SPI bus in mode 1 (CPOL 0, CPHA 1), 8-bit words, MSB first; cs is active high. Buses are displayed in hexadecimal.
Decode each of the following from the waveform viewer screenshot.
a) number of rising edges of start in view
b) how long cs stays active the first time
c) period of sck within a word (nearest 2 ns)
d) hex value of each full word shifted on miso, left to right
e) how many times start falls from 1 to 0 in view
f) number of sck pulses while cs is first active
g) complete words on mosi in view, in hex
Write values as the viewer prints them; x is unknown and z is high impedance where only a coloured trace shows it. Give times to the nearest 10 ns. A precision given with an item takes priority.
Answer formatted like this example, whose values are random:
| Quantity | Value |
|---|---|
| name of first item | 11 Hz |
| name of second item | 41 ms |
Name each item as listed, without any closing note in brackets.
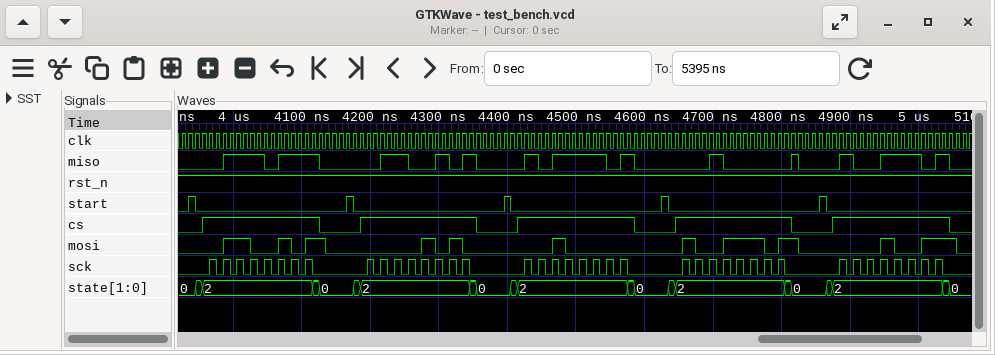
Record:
| Quantity | Value |
|---|---|
| number of rising edges of start in view | 5 |
| how long cs stays active the first time | 170 ns |
| period of sck within a word | 20 ns |
| hex value of each full word shifted on miso, left to right | 77, 65, BD, 20, 9D |
| how many times start falls from 1 to 0 in view | 5 |
| number of sck pulses while cs is first active | 8 |
| complete words on mosi in view, in hex | 65, 0A, 20, 9D, 13 |
